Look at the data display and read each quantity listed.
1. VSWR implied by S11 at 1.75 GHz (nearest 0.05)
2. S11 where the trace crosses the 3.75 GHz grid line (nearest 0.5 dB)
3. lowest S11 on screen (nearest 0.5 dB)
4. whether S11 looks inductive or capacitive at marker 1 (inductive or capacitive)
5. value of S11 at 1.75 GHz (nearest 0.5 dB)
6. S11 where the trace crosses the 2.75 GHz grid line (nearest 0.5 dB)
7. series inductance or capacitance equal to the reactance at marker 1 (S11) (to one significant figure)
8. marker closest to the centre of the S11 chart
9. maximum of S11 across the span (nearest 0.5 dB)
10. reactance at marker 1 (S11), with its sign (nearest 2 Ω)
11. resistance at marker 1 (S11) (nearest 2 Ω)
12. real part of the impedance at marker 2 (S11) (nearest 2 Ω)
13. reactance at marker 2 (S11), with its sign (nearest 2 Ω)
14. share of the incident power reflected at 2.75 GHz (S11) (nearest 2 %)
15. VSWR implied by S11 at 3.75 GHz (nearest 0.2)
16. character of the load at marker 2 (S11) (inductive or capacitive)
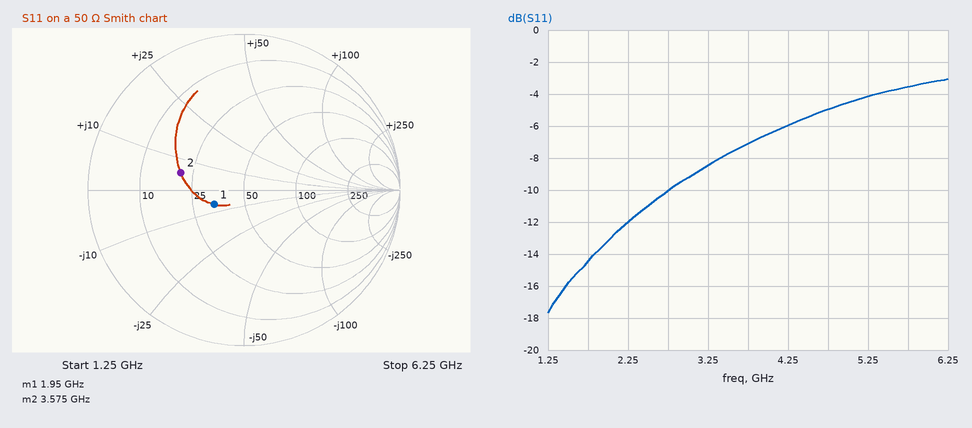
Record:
1.45
-7.0 dB
-17.5 dB
capacitive
-14.5 dB
-10.0 dB
10 pF
marker 1
-3.0 dB
-6 Ω
34 Ω
20 Ω
+6 Ω
10 %
2.6
inductive
